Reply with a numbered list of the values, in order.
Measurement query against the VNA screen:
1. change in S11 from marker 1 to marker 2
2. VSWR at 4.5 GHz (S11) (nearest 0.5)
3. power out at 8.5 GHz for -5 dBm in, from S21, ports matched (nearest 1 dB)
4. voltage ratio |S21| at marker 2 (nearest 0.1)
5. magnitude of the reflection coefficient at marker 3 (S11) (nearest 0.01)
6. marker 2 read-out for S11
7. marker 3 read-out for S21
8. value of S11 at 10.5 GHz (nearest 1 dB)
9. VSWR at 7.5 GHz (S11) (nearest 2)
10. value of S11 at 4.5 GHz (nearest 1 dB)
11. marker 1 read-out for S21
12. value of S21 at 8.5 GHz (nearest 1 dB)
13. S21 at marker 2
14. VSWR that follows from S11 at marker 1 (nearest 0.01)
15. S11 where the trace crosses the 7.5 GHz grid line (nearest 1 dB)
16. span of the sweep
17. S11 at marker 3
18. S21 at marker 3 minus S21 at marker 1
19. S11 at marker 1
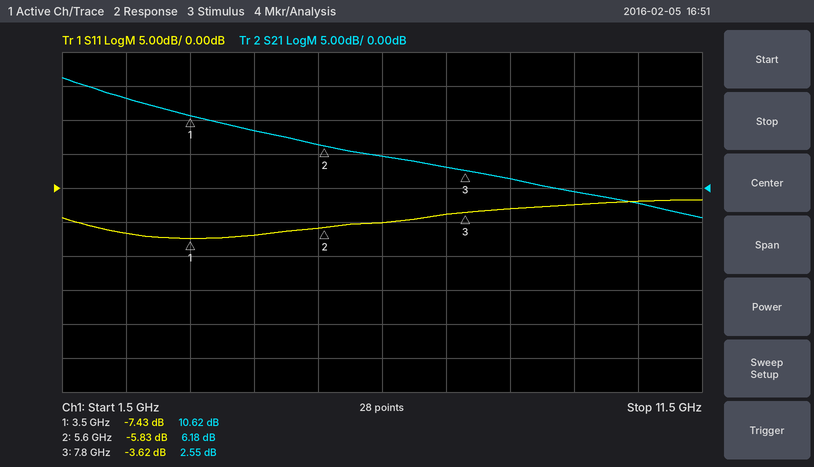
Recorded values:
1. 1.60 dB
2. 2.5
3. -4 dBm
4. 2.0
5. 0.66
6. -5.83 dB
7. 2.55 dB
8. -2 dB
9. 4
10. -7 dB
11. 10.62 dB
12. 1 dB
13. 6.18 dB
14. 2.48
15. -4 dB
16. 10 GHz
17. -3.62 dB
18. -8.07 dB
19. -7.43 dB
